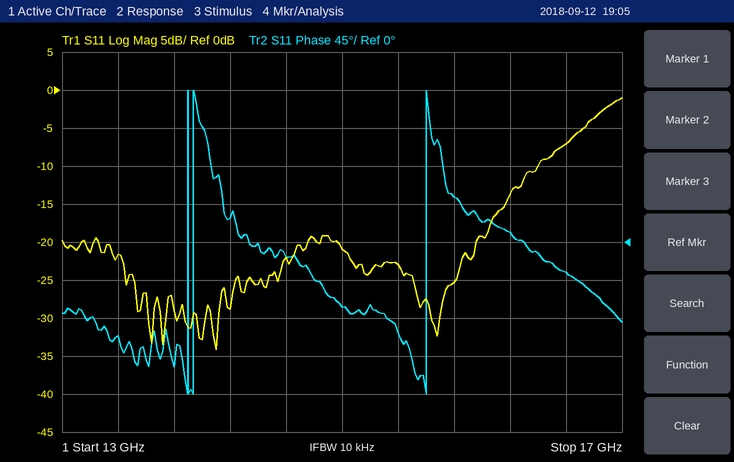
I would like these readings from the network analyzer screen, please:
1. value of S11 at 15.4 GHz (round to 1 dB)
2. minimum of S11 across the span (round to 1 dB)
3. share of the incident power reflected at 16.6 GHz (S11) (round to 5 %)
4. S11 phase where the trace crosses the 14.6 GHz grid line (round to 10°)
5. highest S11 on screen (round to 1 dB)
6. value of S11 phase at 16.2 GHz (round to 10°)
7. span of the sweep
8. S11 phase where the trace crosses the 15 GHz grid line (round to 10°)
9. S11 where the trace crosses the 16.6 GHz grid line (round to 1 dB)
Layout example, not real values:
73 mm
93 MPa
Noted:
-23 dB
-34 dB
20 %
-20°
-1 dB
10°
4 GHz
-80°
-7 dB
